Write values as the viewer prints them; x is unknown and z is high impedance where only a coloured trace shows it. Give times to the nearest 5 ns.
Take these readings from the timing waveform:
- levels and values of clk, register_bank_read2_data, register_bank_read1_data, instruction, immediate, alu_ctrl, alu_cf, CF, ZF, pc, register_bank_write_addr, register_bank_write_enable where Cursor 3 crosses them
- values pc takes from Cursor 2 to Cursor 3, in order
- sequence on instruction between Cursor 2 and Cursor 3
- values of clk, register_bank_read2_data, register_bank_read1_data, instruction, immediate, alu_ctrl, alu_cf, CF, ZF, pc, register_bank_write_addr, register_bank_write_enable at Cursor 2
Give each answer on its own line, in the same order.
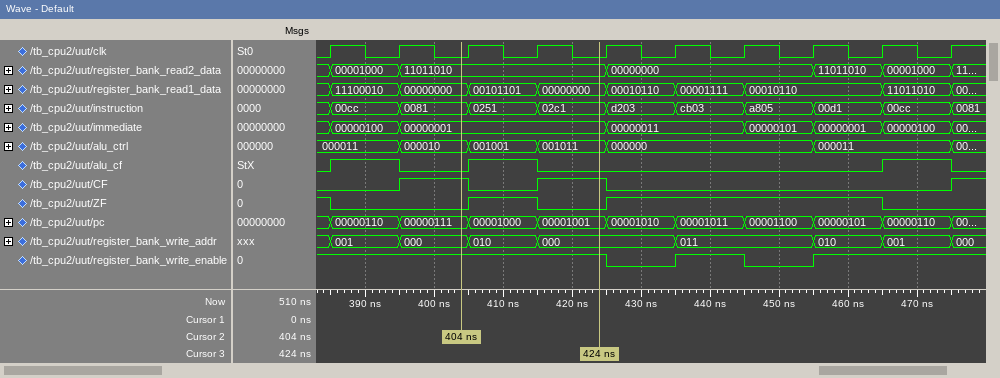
clk=0, register_bank_read2_data=11011010, register_bank_read1_data=00000000, instruction=02c1, immediate=00000001, alu_ctrl=001011, alu_cf=0, CF=1, ZF=0, pc=00001001, register_bank_write_addr=000, register_bank_write_enable=1
00000111, 00001000, 00001001
0081, 0251, 02c1
clk=0, register_bank_read2_data=11011010, register_bank_read1_data=00000000, instruction=0081, immediate=00000001, alu_ctrl=000010, alu_cf=0, CF=1, ZF=0, pc=00000111, register_bank_write_addr=000, register_bank_write_enable=1
